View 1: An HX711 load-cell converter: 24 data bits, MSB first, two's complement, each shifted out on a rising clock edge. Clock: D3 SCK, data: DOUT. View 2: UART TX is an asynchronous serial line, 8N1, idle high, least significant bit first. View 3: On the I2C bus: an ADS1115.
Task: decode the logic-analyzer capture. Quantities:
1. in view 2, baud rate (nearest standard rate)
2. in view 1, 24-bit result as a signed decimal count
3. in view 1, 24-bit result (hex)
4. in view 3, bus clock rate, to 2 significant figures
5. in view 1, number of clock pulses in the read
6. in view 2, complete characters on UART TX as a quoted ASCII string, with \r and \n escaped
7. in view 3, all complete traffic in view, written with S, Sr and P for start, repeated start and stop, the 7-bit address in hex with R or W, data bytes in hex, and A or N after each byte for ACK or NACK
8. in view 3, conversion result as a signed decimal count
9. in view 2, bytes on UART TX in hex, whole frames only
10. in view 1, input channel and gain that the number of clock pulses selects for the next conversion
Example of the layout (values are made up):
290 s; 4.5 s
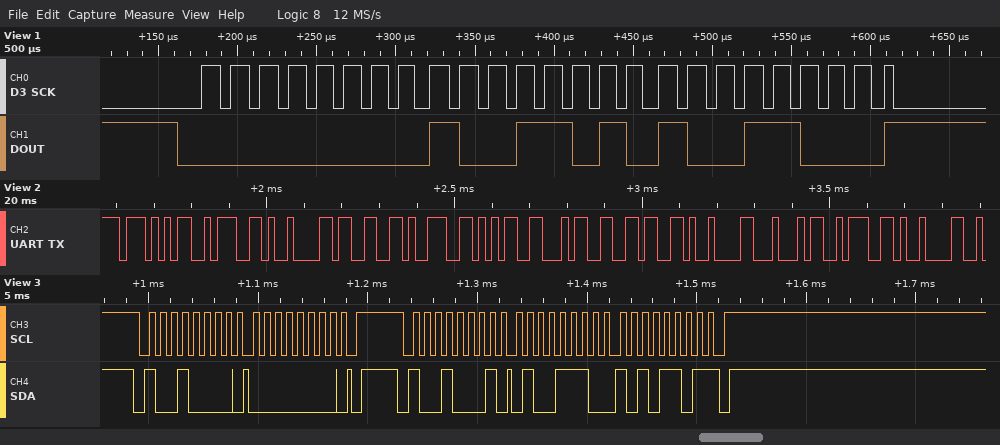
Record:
57600 baud; 39576; 0x009A98; 100 kHz; 25; "W:\t39546\tD:\t"; S 48W A 00 A P S 48R A 4E A AD N P; 20141; 57 3A 09 33 39 35 34 36 09 44 3A 09; channel A, gain 128
